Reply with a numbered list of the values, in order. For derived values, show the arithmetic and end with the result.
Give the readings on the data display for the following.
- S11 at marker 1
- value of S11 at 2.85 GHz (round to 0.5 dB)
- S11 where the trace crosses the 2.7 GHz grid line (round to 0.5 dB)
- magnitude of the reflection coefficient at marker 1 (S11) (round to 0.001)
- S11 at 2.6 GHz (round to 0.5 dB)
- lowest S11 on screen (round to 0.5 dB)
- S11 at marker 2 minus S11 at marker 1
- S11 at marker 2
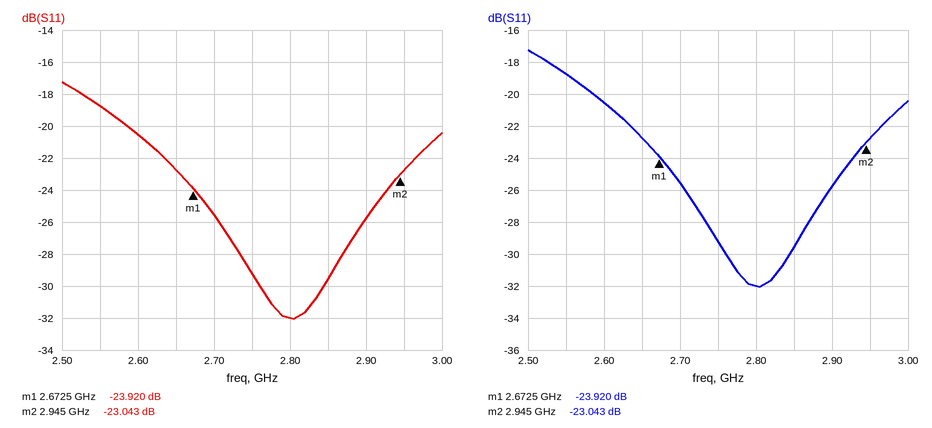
1. -23.920 dB
2. -29.5 dB
3. -25.5 dB
4. 10^(-23.92/20) ≈ 0.064
5. -20.5 dB
6. -32.0 dB
7. -23.043 − (-23.92) = 0.877 dB
8. -23.043 dB
